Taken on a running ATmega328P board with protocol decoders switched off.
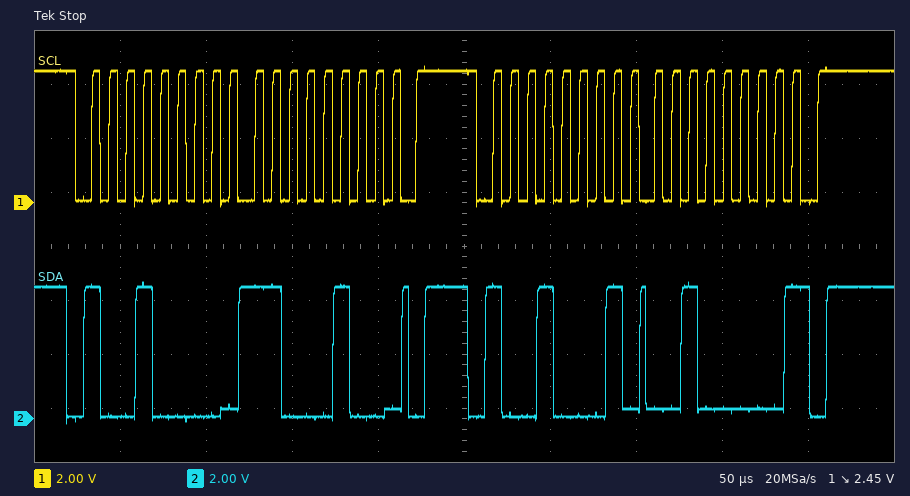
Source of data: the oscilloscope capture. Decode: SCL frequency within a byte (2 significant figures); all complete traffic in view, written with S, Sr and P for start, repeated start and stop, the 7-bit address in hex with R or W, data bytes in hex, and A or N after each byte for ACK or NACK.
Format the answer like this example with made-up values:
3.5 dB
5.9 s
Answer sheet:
100 kHz
S 48W A C4 A P S 48R A 20 N P
